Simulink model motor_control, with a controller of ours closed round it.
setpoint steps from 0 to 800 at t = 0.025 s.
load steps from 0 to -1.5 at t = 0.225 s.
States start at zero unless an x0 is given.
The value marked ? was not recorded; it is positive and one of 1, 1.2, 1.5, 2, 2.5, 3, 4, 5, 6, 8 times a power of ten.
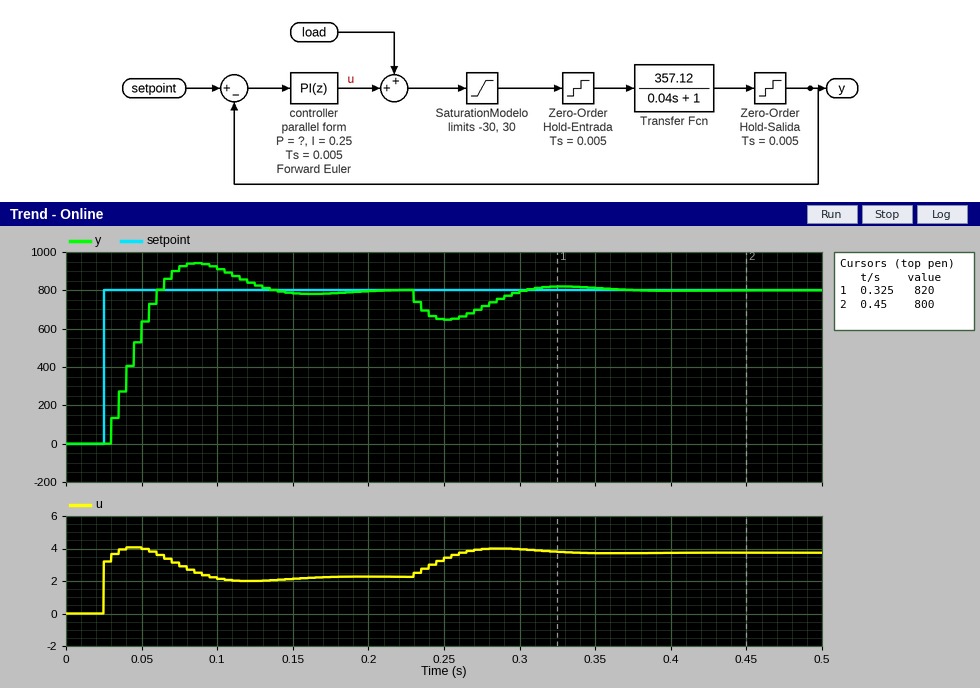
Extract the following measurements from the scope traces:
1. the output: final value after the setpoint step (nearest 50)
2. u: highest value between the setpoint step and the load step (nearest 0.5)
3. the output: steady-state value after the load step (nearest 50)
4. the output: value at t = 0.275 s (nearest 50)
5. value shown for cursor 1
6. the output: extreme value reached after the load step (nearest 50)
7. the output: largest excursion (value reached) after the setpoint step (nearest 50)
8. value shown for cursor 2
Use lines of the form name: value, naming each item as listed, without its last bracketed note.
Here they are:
the output: final value after the setpoint step: 800
u: highest value between the setpoint step and the load step: 4.0
the output: steady-state value after the load step: 800
the output: value at t = 0.275 s: 700
value shown for cursor 1: 820
the output: extreme value reached after the load step: 650
the output: largest excursion (value reached) after the setpoint step: 950
value shown for cursor 2: 800
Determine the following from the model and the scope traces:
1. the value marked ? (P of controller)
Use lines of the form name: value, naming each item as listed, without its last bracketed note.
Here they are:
the value marked ?: 0.004
